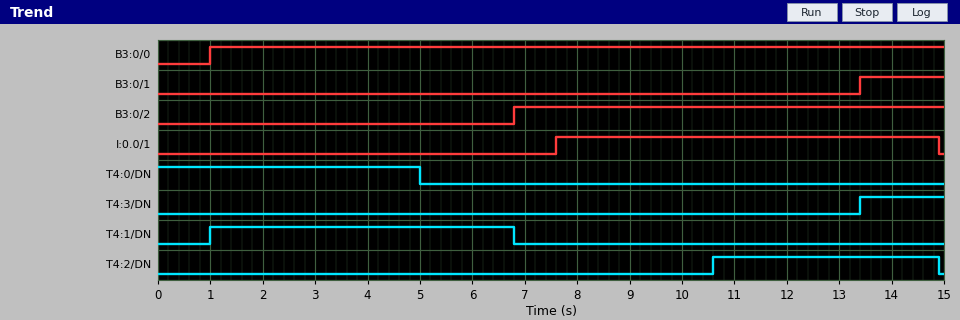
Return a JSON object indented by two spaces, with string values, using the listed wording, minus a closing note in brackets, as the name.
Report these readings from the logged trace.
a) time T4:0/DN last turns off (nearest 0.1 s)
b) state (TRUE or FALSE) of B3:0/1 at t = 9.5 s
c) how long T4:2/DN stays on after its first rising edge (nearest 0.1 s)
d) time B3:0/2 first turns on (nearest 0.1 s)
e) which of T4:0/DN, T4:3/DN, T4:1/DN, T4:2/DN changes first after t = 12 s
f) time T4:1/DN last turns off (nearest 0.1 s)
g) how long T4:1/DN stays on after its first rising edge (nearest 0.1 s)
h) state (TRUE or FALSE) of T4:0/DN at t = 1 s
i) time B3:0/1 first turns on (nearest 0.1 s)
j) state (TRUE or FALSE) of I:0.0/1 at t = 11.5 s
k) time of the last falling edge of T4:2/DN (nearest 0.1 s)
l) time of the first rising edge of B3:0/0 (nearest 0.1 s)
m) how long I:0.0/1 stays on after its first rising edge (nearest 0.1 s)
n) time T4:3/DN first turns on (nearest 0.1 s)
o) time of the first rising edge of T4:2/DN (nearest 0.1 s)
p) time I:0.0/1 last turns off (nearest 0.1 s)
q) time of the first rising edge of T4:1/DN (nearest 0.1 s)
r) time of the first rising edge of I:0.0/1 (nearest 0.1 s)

{
  "time T4:0/DN last turns off": "5.0 s",
  "state (TRUE or FALSE) of B3:0/1 at t = 9.5 s": "FALSE",
  "how long T4:2/DN stays on after its first rising edge": "4.3 s",
  "time B3:0/2 first turns on": "6.8 s",
  "which of T4:0/DN, T4:3/DN, T4:1/DN, T4:2/DN changes first after t = 12 s": "T4:3/DN",
  "time T4:1/DN last turns off": "6.8 s",
  "how long T4:1/DN stays on after its first rising edge": "5.8 s",
  "state (TRUE or FALSE) of T4:0/DN at t = 1 s": "TRUE",
  "time B3:0/1 first turns on": "13.4 s",
  "state (TRUE or FALSE) of I:0.0/1 at t = 11.5 s": "TRUE",
  "time of the last falling edge of T4:2/DN": "14.9 s",
  "time of the first rising edge of B3:0/0": "1.0 s",
  "how long I:0.0/1 stays on after its first rising edge": "7.3 s",
  "time T4:3/DN first turns on": "13.4 s",
  "time of the first rising edge of T4:2/DN": "10.6 s",
  "time I:0.0/1 last turns off": "14.9 s",
  "time of the first rising edge of T4:1/DN": "1.0 s",
  "time of the first rising edge of I:0.0/1": "7.6 s"
}
